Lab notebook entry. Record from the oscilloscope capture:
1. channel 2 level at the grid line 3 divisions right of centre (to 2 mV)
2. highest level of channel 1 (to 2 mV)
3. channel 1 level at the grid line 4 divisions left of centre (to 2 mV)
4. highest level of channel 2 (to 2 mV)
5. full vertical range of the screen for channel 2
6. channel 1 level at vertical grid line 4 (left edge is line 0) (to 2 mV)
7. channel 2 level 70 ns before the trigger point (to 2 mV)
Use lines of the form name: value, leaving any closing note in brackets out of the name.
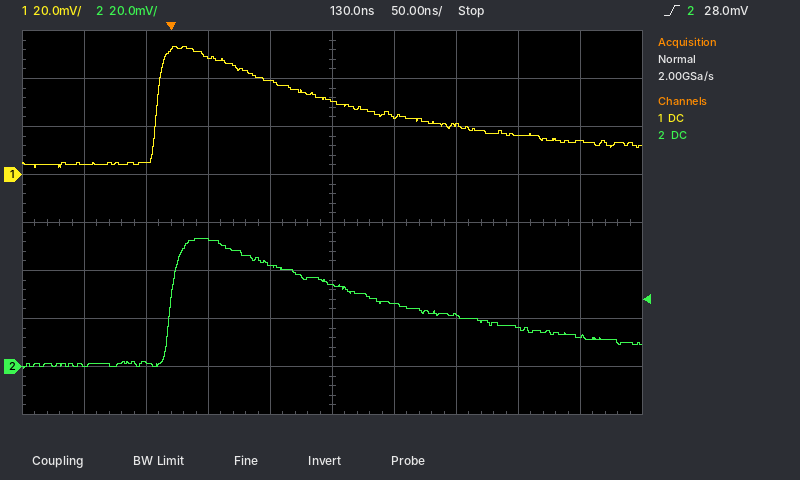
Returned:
channel 2 level at the grid line 3 divisions right of centre: 16 mV
highest level of channel 1: 54 mV
channel 1 level at the grid line 4 divisions left of centre: 4 mV
highest level of channel 2: 54 mV
full vertical range of the screen for channel 2: 160 mV
channel 1 level at vertical grid line 4 (left edge is line 0): 40 mV
channel 2 level 70 ns before the trigger point: 0 mV
